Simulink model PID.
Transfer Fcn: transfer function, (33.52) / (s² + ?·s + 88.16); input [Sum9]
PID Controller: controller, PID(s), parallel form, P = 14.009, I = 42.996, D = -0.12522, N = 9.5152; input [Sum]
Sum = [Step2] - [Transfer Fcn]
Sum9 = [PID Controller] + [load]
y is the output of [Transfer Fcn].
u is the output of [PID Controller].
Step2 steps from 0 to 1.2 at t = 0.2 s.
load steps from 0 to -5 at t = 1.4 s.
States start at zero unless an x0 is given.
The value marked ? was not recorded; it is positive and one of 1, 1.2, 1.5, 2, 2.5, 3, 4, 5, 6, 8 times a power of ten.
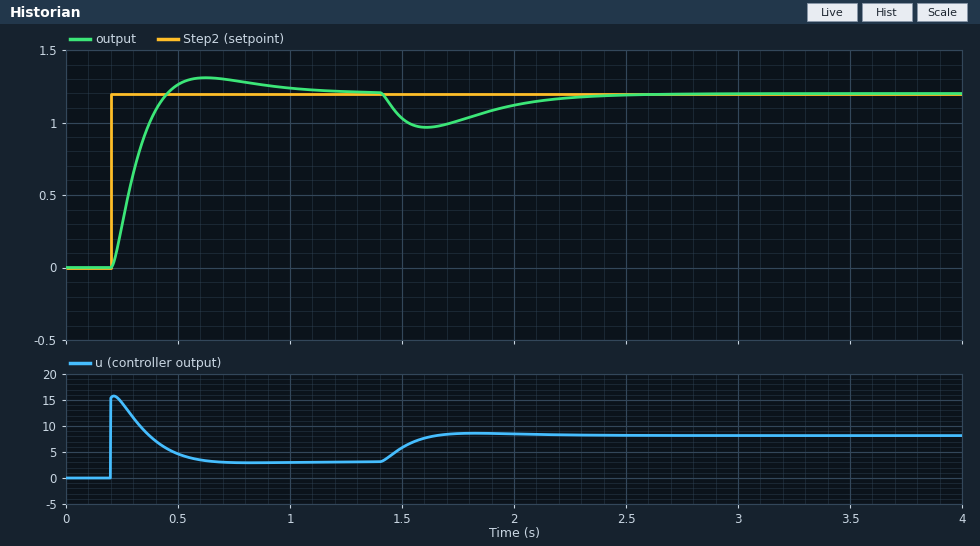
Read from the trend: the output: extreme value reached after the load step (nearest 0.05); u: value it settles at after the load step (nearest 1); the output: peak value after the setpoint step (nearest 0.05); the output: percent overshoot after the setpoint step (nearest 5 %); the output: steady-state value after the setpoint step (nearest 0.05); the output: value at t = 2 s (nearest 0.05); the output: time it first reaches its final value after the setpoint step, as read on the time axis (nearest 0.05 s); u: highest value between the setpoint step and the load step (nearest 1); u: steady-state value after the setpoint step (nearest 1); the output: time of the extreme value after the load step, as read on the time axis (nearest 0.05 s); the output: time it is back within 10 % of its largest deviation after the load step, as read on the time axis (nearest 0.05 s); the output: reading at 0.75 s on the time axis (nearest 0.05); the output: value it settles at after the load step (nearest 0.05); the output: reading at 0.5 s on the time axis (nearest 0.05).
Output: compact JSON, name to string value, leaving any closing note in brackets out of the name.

{"the output: extreme value reached after the load step": "0.95", "u: value it settles at after the load step": "8", "the output: peak value after the setpoint step": "1.30", "the output: percent overshoot after the setpoint step": "10 %", "the output: steady-state value after the setpoint step": "1.20", "the output: value at t = 2 s": "1.10", "the output: time it first reaches its final value after the setpoint step, as read on the time axis": "0.45 s", "u: highest value between the setpoint step and the load step": "16", "u: steady-state value after the setpoint step": "3", "the output: time of the extreme value after the load step, as read on the time axis": "1.60 s", "the output: time it is back within 10 % of its largest deviation after the load step, as read on the time axis": "2.30 s", "the output: reading at 0.75 s on the time axis": "1.30", "the output: value it settles at after the load step": "1.20", "the output: reading at 0.5 s on the time axis": "1.25"}
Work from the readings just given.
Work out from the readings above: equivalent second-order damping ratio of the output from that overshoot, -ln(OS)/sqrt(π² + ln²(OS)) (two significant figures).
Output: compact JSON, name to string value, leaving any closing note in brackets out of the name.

{"equivalent second-order damping ratio of the output from that overshoot, -ln(OS)/sqrt(π² + ln²(OS))": "0.59"}
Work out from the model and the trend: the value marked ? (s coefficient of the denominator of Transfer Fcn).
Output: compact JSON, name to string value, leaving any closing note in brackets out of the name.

{"the value marked ?": "60"}
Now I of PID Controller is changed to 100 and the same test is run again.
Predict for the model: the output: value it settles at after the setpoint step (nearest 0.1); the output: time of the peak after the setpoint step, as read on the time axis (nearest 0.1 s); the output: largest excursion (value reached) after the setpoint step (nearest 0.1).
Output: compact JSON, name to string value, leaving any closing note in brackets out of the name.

{"the output: value it settles at after the setpoint step": "1.2", "the output: time of the peak after the setpoint step, as read on the time axis": "0.5 s", "the output: largest excursion (value reached) after the setpoint step": "1.5"}
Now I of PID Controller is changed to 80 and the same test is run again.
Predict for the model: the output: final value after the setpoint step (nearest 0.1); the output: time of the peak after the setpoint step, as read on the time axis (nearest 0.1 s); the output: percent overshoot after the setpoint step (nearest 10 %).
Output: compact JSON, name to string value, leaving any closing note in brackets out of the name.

{"the output: final value after the setpoint step": "1.2", "the output: time of the peak after the setpoint step, as read on the time axis": "0.5 s", "the output: percent overshoot after the setpoint step": "20 %"}
